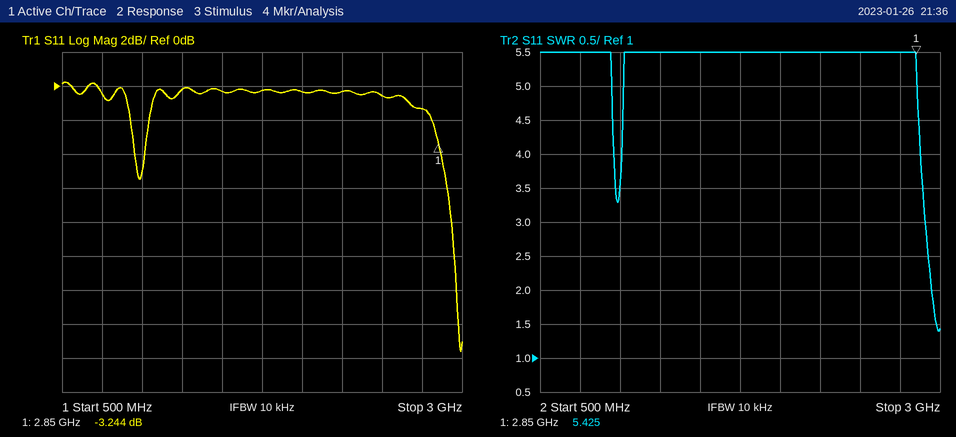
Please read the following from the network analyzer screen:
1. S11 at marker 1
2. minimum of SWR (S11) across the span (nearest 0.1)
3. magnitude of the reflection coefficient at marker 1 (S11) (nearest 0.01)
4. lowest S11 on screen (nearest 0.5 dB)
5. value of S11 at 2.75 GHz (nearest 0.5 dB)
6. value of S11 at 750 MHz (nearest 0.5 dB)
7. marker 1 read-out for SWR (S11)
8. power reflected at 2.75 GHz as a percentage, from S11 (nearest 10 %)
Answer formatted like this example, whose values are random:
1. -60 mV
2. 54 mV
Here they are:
1. -3.244 dB
2. 1.4
3. 0.69
4. -15.5 dB
5. -1.5 dB
6. -0.5 dB
7. 5.425
8. 70 %
